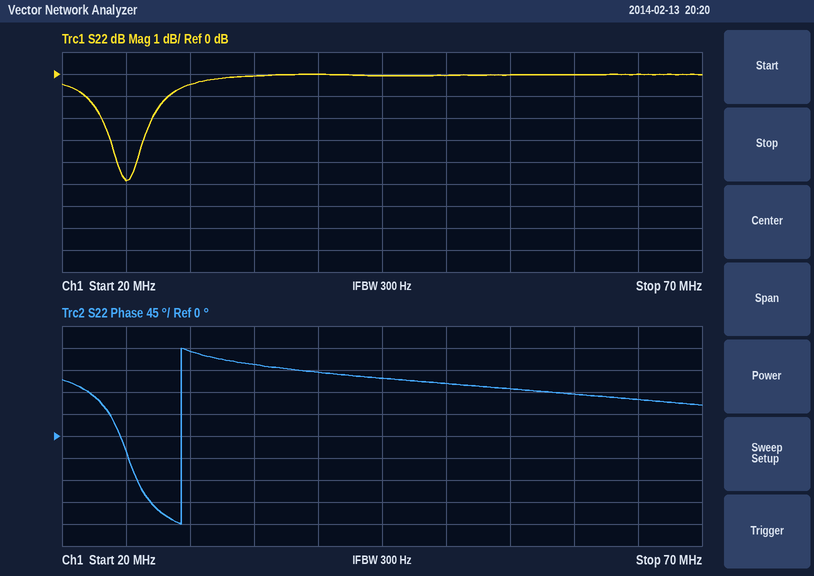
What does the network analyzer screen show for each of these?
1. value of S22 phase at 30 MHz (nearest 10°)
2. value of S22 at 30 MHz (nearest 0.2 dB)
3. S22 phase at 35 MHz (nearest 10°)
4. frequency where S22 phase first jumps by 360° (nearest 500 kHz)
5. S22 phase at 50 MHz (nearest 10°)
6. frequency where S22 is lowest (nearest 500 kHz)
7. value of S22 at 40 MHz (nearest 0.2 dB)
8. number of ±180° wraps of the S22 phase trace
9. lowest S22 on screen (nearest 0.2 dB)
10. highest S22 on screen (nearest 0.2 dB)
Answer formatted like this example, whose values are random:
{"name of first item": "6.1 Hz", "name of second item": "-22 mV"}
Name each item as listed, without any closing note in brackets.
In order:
{"value of S22 phase at 30 MHz": "170°", "value of S22 at 30 MHz": "-0.4 dB", "S22 phase at 35 MHz": "150°", "frequency where S22 phase first jumps by 360°": "29.5 MHz", "S22 phase at 50 MHz": "110°", "frequency where S22 is lowest": "25.0 MHz", "value of S22 at 40 MHz": "0.0 dB", "number of ±180° wraps of the S22 phase trace": "1", "lowest S22 on screen": "-4.8 dB", "highest S22 on screen": "0.0 dB"}
